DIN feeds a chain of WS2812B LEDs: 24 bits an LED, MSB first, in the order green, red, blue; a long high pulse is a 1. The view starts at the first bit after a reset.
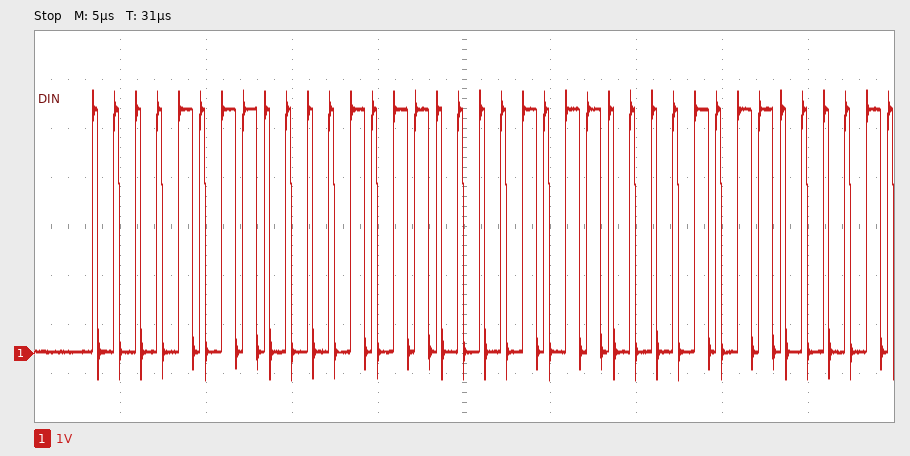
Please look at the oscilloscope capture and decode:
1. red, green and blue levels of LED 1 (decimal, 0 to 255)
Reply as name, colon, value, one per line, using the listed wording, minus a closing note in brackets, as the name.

red, green and blue levels of LED 1: 11, 11, 11
